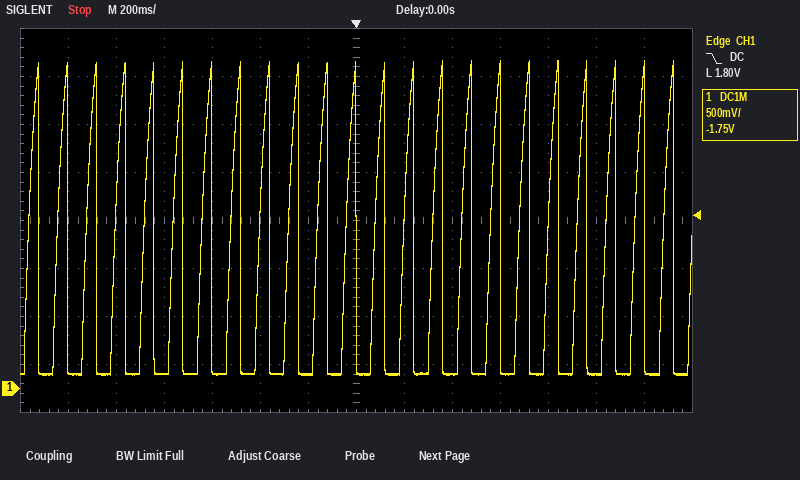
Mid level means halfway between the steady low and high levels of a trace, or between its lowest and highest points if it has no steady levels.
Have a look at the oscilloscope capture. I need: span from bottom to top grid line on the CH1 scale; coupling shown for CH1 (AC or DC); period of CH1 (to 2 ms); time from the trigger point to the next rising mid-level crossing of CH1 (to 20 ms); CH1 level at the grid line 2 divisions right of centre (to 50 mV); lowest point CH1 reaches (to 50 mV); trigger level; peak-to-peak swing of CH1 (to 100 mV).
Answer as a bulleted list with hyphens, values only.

- 4 V
- DC
- 120 ms
- 80 ms
- 150 mV
- 150 mV
- 1.80 V
- 3.30 V
